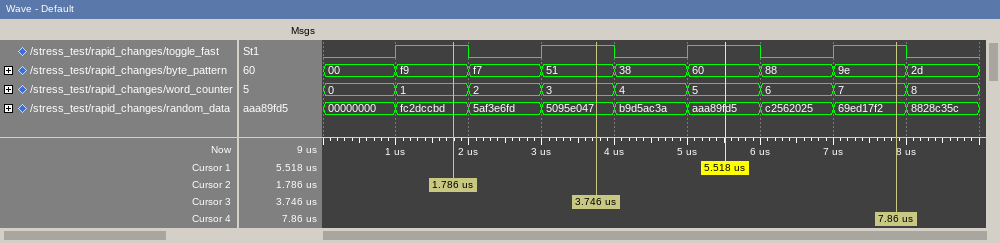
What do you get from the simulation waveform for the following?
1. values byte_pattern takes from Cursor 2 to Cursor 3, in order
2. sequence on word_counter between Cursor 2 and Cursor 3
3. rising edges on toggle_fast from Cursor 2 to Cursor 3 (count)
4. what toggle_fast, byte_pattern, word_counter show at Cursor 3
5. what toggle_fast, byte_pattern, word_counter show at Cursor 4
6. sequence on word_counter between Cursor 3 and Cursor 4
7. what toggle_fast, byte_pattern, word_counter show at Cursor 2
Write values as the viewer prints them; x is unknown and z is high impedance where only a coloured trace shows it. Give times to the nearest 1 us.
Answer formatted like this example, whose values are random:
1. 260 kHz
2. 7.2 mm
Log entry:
1. f9, f7, 51
2. 1, 2, 3
3. 1
4. toggle_fast=1, byte_pattern=51, word_counter=3
5. toggle_fast=1, byte_pattern=9e, word_counter=7
6. 3, 4, 5, 6, 7
7. toggle_fast=1, byte_pattern=f9, word_counter=1
